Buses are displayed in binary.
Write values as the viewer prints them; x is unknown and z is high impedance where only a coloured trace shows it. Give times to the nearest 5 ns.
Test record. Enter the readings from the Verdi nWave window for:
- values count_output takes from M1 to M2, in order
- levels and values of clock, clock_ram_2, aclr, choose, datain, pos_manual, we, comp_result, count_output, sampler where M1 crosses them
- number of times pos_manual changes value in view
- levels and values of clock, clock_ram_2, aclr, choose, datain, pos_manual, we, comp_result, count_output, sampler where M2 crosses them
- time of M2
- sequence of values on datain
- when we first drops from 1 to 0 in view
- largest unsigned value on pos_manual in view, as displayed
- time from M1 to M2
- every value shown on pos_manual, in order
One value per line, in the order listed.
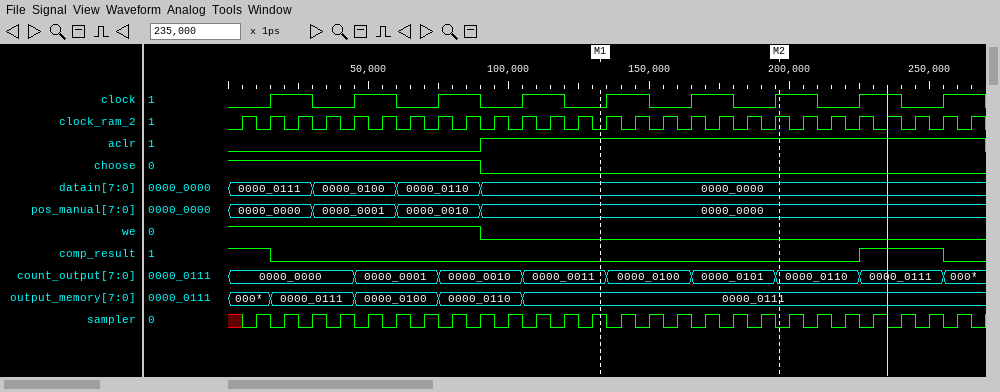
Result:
0000_0011, 0000_0100, 0000_0101, 0000_0110
clock=0, clock_ram_2=0, aclr=1, choose=0, datain=0000_0000, pos_manual=0000_0000, we=0, comp_result=0, count_output=0000_0011, sampler=1
3
clock=1, clock_ram_2=1, aclr=1, choose=0, datain=0000_0000, pos_manual=0000_0000, we=0, comp_result=0, count_output=0000_0110, sampler=0
195 ns
0000_0111, 0000_0100, 0000_0110, 0000_0000
90 ns
0000_0010
65 ns
0000_0000, 0000_0001, 0000_0010, 0000_0000
